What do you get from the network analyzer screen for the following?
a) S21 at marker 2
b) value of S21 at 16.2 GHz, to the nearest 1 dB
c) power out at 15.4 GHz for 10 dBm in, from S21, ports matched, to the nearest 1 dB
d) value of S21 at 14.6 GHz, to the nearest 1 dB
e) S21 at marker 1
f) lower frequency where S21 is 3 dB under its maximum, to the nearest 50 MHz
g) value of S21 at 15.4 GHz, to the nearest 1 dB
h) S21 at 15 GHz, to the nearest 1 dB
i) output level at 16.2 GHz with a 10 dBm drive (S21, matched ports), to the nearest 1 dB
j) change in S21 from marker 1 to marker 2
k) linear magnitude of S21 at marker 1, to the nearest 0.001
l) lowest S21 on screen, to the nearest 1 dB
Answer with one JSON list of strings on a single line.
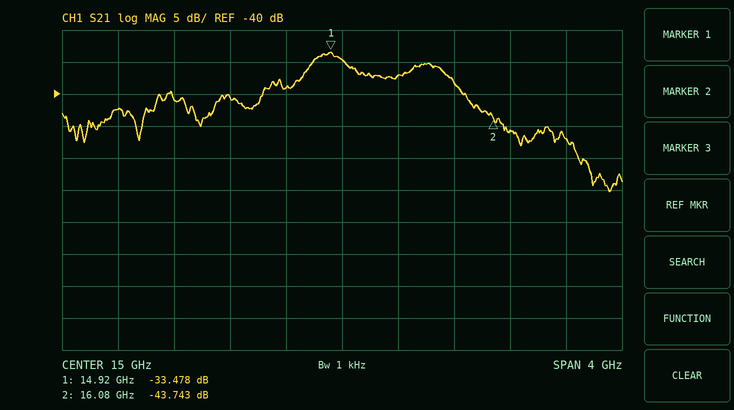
["-43.743 dB", "-46 dB", "-27 dBm", "-39 dB", "-33.478 dB", "14.75 GHz", "-37 dB", "-35 dB", "-36 dBm", "-10.265 dB", "0.021", "-55 dB"]
